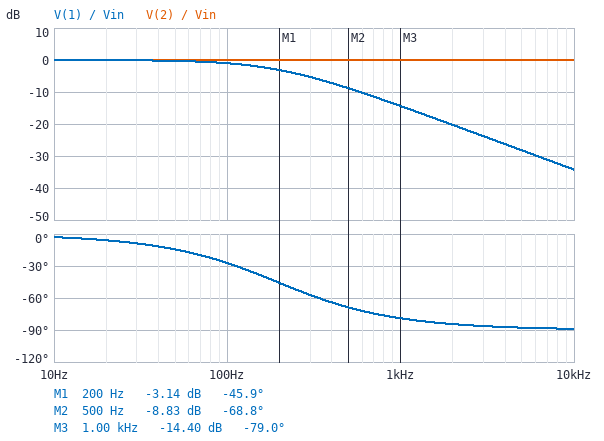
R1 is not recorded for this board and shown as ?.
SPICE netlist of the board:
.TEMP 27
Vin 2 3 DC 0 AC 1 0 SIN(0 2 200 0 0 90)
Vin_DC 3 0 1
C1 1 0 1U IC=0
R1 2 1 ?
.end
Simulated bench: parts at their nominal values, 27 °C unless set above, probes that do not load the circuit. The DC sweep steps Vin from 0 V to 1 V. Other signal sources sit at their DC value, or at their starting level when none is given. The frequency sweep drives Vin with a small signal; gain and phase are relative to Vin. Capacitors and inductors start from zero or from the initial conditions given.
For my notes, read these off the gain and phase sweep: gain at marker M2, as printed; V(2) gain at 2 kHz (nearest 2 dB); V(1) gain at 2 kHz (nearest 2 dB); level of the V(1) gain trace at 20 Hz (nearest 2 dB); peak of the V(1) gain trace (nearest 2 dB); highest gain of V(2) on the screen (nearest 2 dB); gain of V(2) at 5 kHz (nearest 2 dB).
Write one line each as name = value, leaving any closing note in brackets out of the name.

gain at marker M2, as printed = -8.83 dB
V(2) gain at 2 kHz = 0 dB
V(1) gain at 2 kHz = -20 dB
level of the V(1) gain trace at 20 Hz = 0 dB
peak of the V(1) gain trace = 0 dB
highest gain of V(2) on the screen = 0 dB
gain of V(2) at 5 kHz = 0 dB
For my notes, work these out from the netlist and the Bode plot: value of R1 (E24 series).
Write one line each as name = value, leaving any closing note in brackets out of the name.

value of R1 = 820 Ω
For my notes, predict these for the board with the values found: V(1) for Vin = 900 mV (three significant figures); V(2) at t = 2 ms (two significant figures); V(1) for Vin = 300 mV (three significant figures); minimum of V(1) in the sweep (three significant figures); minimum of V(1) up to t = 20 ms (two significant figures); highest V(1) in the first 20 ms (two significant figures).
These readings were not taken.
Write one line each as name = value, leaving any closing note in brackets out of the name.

V(1) for Vin = 900 mV = 1.90 V
V(2) at t = 2 ms = -620 mV
V(1) for Vin = 300 mV = 1.30 V
minimum of V(1) in the sweep = 1.00 V
minimum of V(1) up to t = 20 ms = -440 mV
highest V(1) in the first 20 ms = 2.4 V
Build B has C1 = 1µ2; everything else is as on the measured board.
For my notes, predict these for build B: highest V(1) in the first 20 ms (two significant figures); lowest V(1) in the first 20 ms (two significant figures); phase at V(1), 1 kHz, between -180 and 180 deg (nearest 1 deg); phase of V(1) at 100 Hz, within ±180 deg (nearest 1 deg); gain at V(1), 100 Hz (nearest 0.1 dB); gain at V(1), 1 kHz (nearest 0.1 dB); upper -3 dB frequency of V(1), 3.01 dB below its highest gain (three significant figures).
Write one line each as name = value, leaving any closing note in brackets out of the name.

highest V(1) in the first 20 ms = 2.3 V
lowest V(1) in the first 20 ms = -330 mV
phase at V(1), 1 kHz, between -180 and 180 deg = -81 deg
phase of V(1) at 100 Hz, within ±180 deg = -32 deg
gain at V(1), 100 Hz = -1.4 dB
gain at V(1), 1 kHz = -15.9 dB
upper -3 dB frequency of V(1), 3.01 dB below its highest gain = 162 Hz
